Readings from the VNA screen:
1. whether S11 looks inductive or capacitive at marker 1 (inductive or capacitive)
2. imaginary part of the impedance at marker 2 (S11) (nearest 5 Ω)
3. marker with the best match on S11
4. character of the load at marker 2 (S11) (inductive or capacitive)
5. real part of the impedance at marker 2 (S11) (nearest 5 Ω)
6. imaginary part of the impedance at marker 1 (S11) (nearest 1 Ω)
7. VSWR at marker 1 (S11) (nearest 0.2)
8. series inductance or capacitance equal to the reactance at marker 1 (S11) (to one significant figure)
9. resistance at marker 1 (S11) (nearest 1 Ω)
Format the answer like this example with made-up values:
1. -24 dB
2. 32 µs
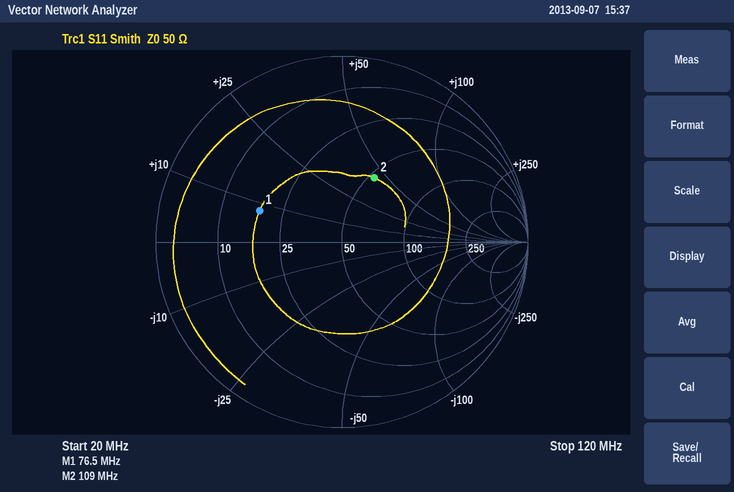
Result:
1. inductive
2. +45 Ω
3. marker 2
4. inductive
5. 55 Ω
6. +8 Ω
7. 2.8
8. 20 nH
9. 18 Ω
